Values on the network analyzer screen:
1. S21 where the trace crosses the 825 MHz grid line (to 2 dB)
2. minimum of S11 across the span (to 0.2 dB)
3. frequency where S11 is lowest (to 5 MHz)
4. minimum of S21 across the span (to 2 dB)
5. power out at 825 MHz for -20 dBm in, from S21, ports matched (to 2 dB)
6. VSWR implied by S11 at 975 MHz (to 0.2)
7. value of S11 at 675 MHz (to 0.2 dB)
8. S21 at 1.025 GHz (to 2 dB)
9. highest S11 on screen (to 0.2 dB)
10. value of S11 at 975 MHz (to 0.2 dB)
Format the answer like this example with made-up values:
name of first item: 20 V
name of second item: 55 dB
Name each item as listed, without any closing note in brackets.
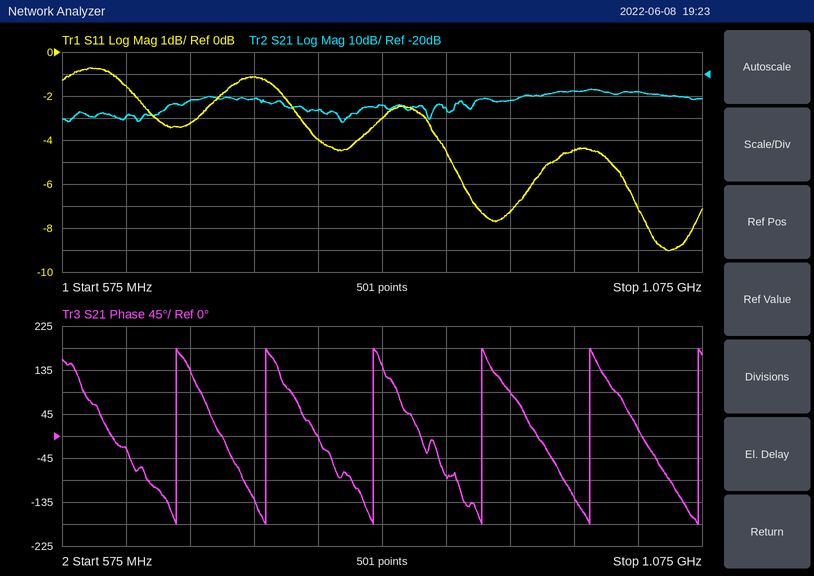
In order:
S21 where the trace crosses the 825 MHz grid line: -34 dB
minimum of S11 across the span: -9.0 dB
frequency where S11 is lowest: 1.050 GHz
minimum of S21 across the span: -42 dB
power out at 825 MHz for -20 dBm in, from S21, ports matched: -54 dBm
VSWR implied by S11 at 975 MHz: 4.0
value of S11 at 675 MHz: -3.2 dB
S21 at 1.025 GHz: -28 dB
highest S11 on screen: -0.8 dB
value of S11 at 975 MHz: -4.4 dB
